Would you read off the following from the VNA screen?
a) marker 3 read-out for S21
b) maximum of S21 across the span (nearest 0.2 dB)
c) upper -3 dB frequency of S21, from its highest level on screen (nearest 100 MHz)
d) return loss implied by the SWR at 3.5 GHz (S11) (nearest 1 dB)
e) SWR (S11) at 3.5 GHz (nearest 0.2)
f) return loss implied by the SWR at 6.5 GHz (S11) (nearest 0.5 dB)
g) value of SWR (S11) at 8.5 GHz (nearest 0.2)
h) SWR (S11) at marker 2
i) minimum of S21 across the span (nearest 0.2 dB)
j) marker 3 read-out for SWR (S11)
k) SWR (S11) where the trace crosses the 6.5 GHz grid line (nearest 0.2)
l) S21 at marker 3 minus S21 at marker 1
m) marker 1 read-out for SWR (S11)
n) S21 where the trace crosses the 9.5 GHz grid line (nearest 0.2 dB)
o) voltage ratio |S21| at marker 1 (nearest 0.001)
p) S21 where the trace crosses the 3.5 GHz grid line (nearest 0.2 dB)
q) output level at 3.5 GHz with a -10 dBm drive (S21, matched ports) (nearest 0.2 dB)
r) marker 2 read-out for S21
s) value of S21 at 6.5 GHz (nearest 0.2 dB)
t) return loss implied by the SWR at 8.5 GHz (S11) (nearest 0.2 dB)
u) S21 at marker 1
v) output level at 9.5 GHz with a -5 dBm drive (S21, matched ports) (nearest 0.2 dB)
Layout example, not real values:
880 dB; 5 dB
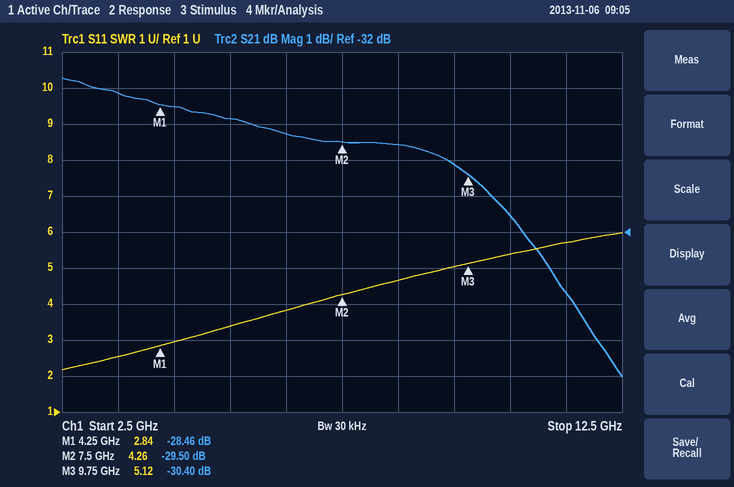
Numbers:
-30.40 dB; -27.8 dB; 10.0 GHz; 7 dB; 2.6; 4.5 dB; 4.6; 4.26; -36.0 dB; 5.12; 3.8; -1.94 dB; 2.84; -30.2 dB; 0.038; -28.2 dB; -38.2 dBm; -29.50 dB; -29.2 dB; 3.8 dB; -28.46 dB; -35.2 dBm
